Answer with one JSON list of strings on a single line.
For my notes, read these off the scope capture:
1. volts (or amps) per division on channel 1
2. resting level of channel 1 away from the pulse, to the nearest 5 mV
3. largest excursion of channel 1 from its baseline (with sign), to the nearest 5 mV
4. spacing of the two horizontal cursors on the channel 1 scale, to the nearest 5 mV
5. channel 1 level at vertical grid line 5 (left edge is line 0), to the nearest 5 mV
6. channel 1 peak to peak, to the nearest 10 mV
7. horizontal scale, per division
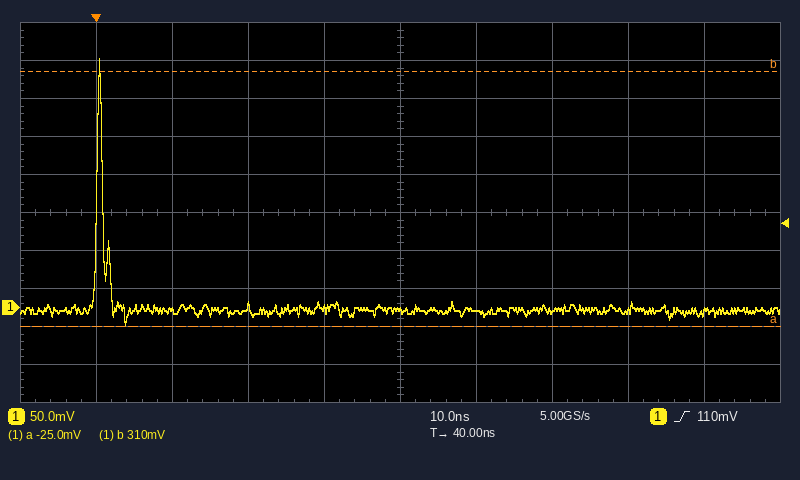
["50 mV", "-5 mV", "+330 mV", "335 mV", "-5 mV", "350 mV", "10 ns"]
